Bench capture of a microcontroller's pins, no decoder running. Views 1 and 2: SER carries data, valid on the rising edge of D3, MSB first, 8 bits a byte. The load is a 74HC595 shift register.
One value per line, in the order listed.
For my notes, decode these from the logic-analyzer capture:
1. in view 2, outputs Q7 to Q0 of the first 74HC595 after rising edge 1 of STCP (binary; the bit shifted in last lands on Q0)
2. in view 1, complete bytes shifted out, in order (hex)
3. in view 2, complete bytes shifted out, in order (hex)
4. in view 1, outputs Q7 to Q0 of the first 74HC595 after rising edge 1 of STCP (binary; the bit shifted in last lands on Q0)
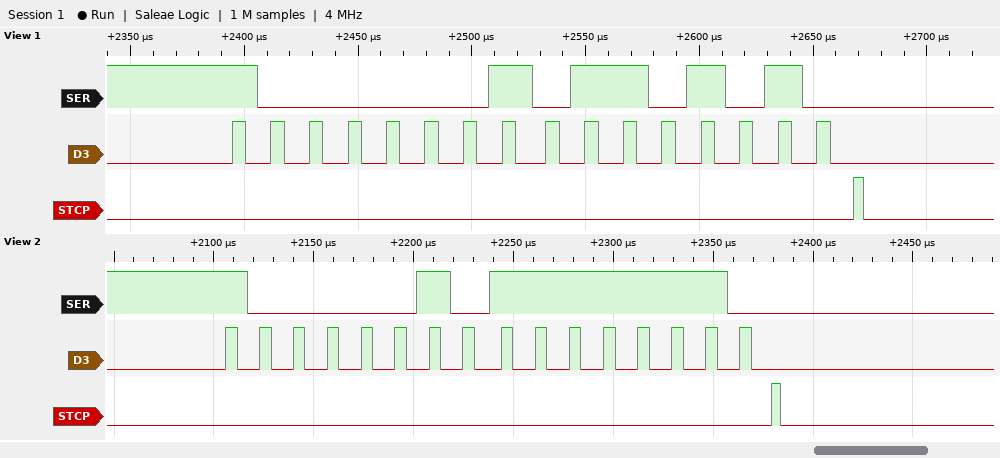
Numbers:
11111110
81 6A
82 FE
01101010
